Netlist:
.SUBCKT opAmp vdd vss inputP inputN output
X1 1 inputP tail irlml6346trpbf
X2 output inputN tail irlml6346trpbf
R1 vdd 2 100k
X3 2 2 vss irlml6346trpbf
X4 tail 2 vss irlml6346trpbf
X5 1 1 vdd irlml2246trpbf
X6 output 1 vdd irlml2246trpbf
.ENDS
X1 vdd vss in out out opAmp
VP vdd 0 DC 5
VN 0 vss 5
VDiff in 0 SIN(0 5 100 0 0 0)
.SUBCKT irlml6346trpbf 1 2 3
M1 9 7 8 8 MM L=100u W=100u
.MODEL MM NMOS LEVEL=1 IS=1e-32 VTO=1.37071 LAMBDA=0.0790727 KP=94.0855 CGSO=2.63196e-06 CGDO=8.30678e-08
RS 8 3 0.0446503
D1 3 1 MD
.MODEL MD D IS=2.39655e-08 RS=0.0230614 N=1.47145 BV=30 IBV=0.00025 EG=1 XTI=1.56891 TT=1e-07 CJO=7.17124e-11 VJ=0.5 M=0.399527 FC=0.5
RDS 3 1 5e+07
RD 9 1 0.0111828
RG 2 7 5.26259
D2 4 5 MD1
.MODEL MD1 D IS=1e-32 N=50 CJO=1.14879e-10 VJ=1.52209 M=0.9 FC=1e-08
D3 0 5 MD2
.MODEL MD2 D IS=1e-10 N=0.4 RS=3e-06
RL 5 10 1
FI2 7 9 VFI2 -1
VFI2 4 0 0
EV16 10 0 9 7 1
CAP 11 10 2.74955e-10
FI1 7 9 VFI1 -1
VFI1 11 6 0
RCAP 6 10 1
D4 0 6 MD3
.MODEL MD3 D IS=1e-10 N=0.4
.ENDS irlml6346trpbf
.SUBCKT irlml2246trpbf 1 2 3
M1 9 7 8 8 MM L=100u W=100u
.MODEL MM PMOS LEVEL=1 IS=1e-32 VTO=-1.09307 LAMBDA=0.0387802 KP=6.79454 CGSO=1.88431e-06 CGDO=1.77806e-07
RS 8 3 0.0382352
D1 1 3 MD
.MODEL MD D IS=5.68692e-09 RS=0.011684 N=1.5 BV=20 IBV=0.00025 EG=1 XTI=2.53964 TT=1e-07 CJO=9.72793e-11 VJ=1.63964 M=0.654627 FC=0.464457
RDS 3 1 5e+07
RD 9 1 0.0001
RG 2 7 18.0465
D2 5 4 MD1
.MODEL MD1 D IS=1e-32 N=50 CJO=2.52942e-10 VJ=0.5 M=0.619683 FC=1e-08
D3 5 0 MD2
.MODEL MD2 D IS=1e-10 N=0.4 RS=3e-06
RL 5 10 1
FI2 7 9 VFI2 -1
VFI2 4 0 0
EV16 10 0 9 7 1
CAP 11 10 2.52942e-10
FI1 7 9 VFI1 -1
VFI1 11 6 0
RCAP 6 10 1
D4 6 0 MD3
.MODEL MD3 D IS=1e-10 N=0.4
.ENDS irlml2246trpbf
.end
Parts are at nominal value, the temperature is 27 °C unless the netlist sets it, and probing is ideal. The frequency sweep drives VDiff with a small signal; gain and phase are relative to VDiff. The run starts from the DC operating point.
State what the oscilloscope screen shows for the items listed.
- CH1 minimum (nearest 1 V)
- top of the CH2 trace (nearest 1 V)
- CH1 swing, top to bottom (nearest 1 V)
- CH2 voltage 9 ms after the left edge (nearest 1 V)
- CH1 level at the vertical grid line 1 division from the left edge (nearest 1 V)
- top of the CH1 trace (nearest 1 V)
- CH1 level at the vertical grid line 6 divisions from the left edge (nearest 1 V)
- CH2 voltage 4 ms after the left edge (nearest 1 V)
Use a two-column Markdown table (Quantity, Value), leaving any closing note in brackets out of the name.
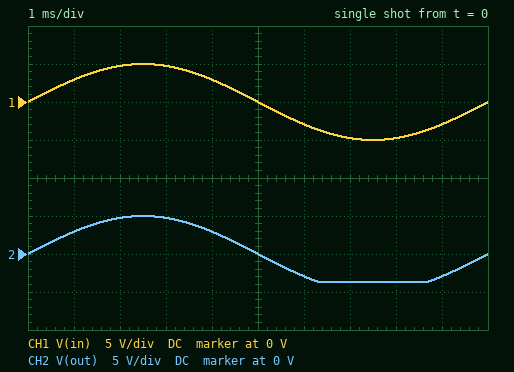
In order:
| Quantity | Value |
|---|---|
| CH1 minimum | -5 V |
| top of the CH2 trace | 5 V |
| CH1 swing, top to bottom | 10 V |
| CH2 voltage 9 ms after the left edge | -3 V |
| CH1 level at the vertical grid line 1 division from the left edge | 3 V |
| top of the CH1 trace | 5 V |
| CH1 level at the vertical grid line 6 divisions from the left edge | -3 V |
| CH2 voltage 4 ms after the left edge | 3 V |
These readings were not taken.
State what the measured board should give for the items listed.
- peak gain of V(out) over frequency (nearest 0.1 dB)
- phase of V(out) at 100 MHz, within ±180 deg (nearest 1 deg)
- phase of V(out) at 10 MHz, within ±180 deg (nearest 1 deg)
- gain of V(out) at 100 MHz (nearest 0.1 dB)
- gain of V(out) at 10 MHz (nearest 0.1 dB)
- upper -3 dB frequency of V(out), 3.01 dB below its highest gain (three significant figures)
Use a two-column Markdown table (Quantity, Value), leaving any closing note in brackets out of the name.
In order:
| Quantity | Value |
|---|---|
| peak gain of V(out) over frequency | 0.4 dB |
| phase of V(out) at 100 MHz, within ±180 deg | -38 deg |
| phase of V(out) at 10 MHz, within ±180 deg | -16 deg |
| gain of V(out) at 100 MHz | -7.8 dB |
| gain of V(out) at 10 MHz | 0.4 dB |
| upper -3 dB frequency of V(out), 3.01 dB below its highest gain | 23.1 MHz |
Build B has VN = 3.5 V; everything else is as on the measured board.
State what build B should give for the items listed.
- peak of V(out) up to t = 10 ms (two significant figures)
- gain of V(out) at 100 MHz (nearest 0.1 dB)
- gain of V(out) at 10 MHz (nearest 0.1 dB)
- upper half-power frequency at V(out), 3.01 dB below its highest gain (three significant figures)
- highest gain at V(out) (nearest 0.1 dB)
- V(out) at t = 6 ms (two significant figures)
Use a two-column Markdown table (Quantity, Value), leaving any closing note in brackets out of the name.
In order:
| Quantity | Value |
|---|---|
| peak of V(out) up to t = 10 ms | 5.0 V |
| gain of V(out) at 100 MHz | -8.5 dB |
| gain of V(out) at 10 MHz | 0.5 dB |
| upper half-power frequency at V(out), 3.01 dB below its highest gain | 19.1 MHz |
| highest gain at V(out) | 0.6 dB |
| V(out) at t = 6 ms | -2.1 V |
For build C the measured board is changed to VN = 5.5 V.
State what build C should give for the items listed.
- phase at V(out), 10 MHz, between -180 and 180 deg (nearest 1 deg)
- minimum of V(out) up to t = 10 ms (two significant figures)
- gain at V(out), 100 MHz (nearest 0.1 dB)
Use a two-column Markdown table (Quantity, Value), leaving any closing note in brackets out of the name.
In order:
| Quantity | Value |
|---|---|
| phase at V(out), 10 MHz, between -180 and 180 deg | -15 deg |
| minimum of V(out) up to t = 10 ms | -4.1 V |
| gain at V(out), 100 MHz | -7.6 dB |
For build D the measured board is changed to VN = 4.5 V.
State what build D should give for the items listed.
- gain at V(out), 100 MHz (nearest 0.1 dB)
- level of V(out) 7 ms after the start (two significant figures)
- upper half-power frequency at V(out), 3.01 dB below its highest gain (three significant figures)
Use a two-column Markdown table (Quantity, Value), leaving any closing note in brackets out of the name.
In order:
| Quantity | Value |
|---|---|
| gain at V(out), 100 MHz | -8.0 dB |
| level of V(out) 7 ms after the start | -3.1 V |
| upper half-power frequency at V(out), 3.01 dB below its highest gain | 21.8 MHz |
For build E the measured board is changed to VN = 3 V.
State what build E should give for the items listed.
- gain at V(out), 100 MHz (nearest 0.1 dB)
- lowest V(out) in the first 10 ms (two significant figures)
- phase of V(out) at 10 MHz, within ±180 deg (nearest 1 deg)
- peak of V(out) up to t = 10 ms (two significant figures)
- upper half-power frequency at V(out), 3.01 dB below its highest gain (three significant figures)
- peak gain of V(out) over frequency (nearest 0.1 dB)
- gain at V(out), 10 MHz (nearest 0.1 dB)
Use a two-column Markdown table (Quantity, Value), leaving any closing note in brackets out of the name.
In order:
| Quantity | Value |
|---|---|
| gain at V(out), 100 MHz | -8.9 dB |
| lowest V(out) in the first 10 ms | -1.6 V |
| phase of V(out) at 10 MHz, within ±180 deg | -25 deg |
| peak of V(out) up to t = 10 ms | 5.0 V |
| upper half-power frequency at V(out), 3.01 dB below its highest gain | 17.6 MHz |
| peak gain of V(out) over frequency | 0.7 dB |
| gain at V(out), 10 MHz | 0.6 dB |
